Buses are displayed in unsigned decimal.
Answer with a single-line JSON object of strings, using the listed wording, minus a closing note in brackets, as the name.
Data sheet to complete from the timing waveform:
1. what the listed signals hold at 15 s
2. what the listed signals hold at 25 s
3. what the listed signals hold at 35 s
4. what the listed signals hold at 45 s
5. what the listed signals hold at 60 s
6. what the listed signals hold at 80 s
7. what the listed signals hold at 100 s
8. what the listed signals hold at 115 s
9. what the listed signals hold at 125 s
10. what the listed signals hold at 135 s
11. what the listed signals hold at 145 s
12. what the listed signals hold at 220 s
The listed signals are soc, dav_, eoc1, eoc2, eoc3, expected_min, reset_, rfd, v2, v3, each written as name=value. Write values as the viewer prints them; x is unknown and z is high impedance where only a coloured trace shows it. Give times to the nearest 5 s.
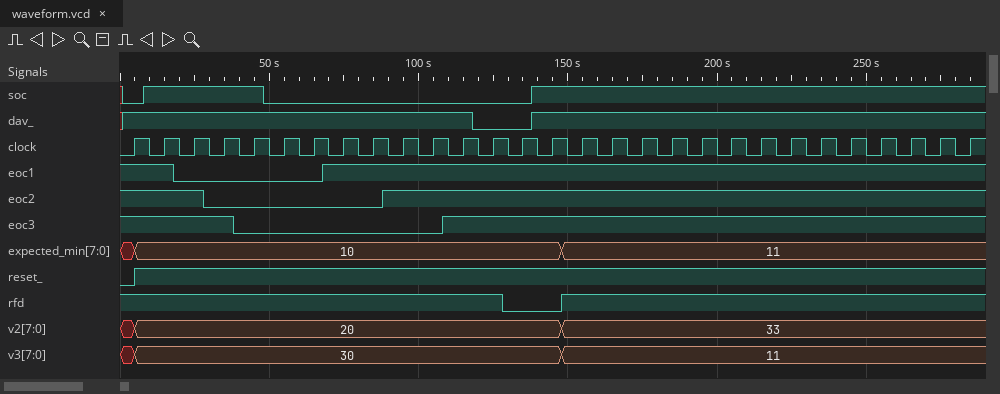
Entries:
{"what the listed signals hold at 15 s": "soc=1, dav_=1, eoc1=1, eoc2=1, eoc3=1, expected_min=10, reset_=1, rfd=1, v2=20, v3=30", "what the listed signals hold at 25 s": "soc=1, dav_=1, eoc1=0, eoc2=1, eoc3=1, expected_min=10, reset_=1, rfd=1, v2=20, v3=30", "what the listed signals hold at 35 s": "soc=1, dav_=1, eoc1=0, eoc2=0, eoc3=1, expected_min=10, reset_=1, rfd=1, v2=20, v3=30", "what the listed signals hold at 45 s": "soc=1, dav_=1, eoc1=0, eoc2=0, eoc3=0, expected_min=10, reset_=1, rfd=1, v2=20, v3=30", "what the listed signals hold at 60 s": "soc=0, dav_=1, eoc1=0, eoc2=0, eoc3=0, expected_min=10, reset_=1, rfd=1, v2=20, v3=30", "what the listed signals hold at 80 s": "soc=0, dav_=1, eoc1=1, eoc2=0, eoc3=0, expected_min=10, reset_=1, rfd=1, v2=20, v3=30", "what the listed signals hold at 100 s": "soc=0, dav_=1, eoc1=1, eoc2=1, eoc3=0, expected_min=10, reset_=1, rfd=1, v2=20, v3=30", "what the listed signals hold at 115 s": "soc=0, dav_=1, eoc1=1, eoc2=1, eoc3=1, expected_min=10, reset_=1, rfd=1, v2=20, v3=30", "what the listed signals hold at 125 s": "soc=0, dav_=0, eoc1=1, eoc2=1, eoc3=1, expected_min=10, reset_=1, rfd=1, v2=20, v3=30", "what the listed signals hold at 135 s": "soc=0, dav_=0, eoc1=1, eoc2=1, eoc3=1, expected_min=10, reset_=1, rfd=0, v2=20, v3=30", "what the listed signals hold at 145 s": "soc=1, dav_=1, eoc1=1, eoc2=1, eoc3=1, expected_min=10, reset_=1, rfd=0, v2=20, v3=30", "what the listed signals hold at 220 s": "soc=1, dav_=1, eoc1=1, eoc2=1, eoc3=1, expected_min=11, reset_=1, rfd=1, v2=33, v3=11"}
